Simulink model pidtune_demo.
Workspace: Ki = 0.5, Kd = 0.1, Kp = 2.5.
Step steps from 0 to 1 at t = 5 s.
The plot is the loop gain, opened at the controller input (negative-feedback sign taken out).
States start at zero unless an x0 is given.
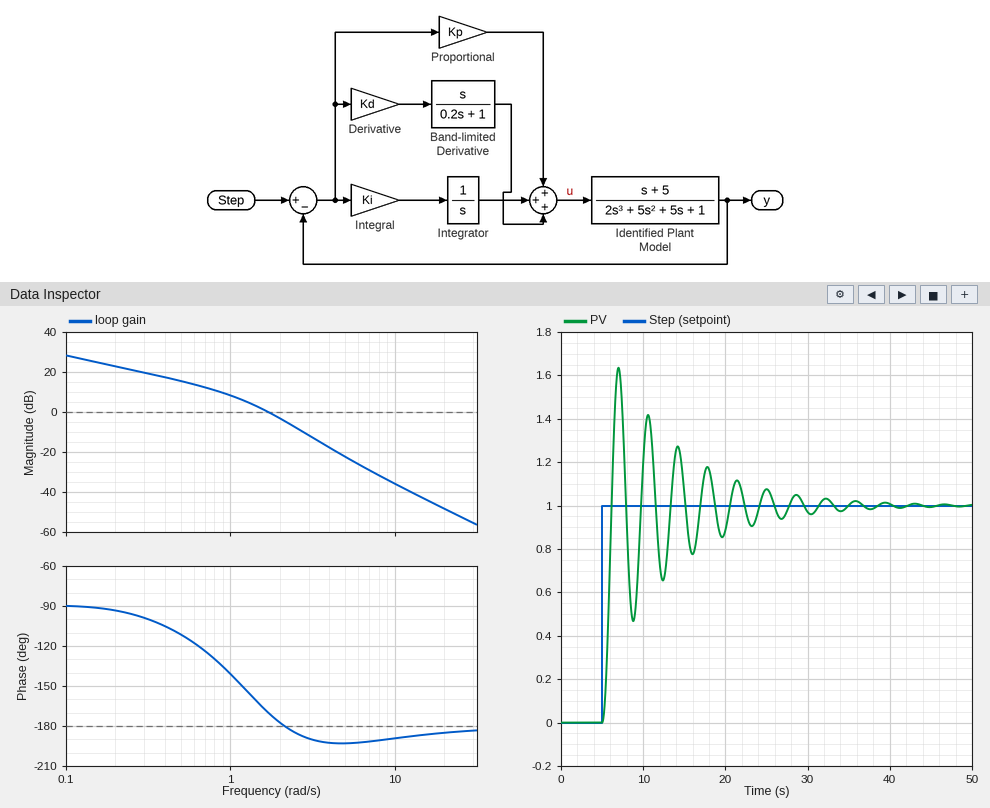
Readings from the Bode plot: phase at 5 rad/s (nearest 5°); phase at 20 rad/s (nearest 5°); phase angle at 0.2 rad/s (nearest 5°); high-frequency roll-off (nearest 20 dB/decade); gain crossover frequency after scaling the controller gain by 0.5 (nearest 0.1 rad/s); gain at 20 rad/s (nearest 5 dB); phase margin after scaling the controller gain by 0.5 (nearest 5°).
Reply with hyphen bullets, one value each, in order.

- -195°
- -185°
- -95°
- -40 dB/decade
- 1.2 rad/s
- -50 dB
- 30°
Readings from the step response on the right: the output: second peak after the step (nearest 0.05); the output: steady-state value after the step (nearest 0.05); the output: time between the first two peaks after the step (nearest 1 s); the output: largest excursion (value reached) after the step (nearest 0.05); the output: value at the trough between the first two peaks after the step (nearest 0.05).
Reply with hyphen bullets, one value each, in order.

- 1.40
- 1.00
- 4 s
- 1.65
- 0.45
